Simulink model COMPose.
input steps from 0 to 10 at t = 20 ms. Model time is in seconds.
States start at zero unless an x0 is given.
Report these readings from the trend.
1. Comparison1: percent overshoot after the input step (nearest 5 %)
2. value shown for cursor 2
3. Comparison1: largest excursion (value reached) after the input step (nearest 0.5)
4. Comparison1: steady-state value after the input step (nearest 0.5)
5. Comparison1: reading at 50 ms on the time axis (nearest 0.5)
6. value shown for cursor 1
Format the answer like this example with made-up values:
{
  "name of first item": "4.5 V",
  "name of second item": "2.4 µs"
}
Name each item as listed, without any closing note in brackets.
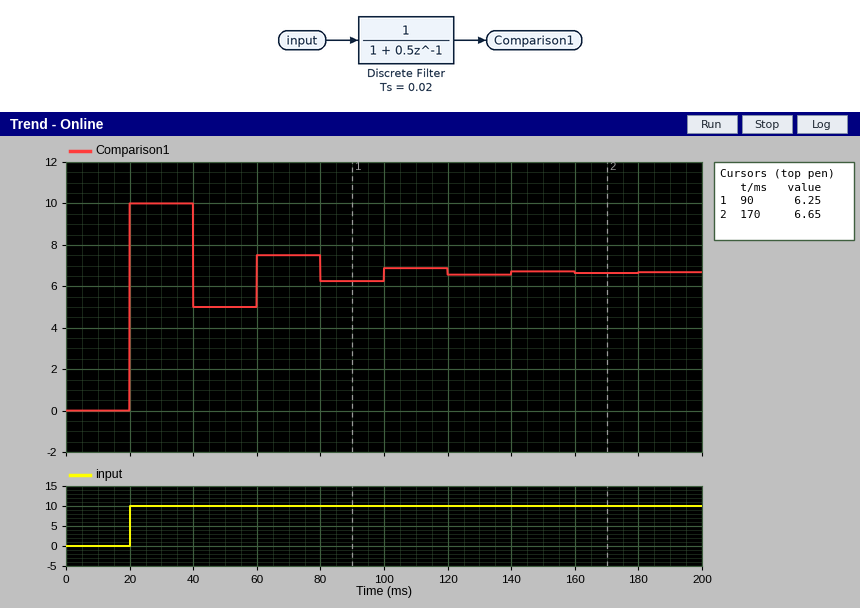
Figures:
{
  "Comparison1: percent overshoot after the input step": "50 %",
  "value shown for cursor 2": "6.65",
  "Comparison1: largest excursion (value reached) after the input step": "10.0",
  "Comparison1: steady-state value after the input step": "6.5",
  "Comparison1: reading at 50 ms on the time axis": "5.0",
  "value shown for cursor 1": "6.25"
}
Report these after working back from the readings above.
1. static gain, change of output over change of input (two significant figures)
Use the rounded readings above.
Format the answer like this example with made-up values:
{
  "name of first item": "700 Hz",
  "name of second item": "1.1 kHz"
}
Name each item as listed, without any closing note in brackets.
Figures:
{
  "static gain, change of output over change of input": "0.65"
}
